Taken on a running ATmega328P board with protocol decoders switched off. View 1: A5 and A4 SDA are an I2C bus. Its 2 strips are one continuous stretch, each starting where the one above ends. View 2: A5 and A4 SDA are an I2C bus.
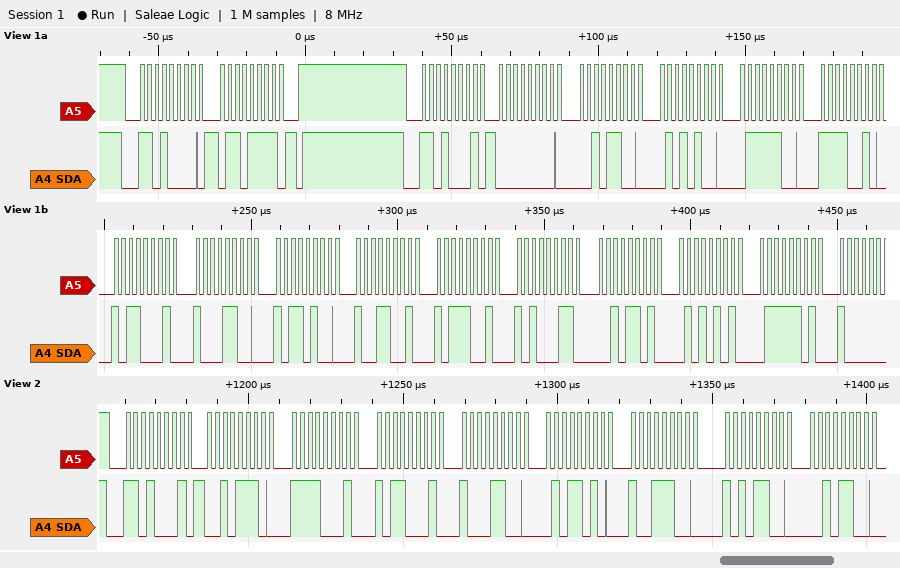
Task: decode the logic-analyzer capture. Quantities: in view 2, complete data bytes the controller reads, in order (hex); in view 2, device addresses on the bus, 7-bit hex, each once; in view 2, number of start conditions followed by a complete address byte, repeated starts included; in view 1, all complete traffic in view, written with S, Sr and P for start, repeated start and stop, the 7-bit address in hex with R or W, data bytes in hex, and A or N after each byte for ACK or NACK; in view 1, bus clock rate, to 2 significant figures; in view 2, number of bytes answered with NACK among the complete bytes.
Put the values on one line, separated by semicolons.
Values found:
2E F1 B1 8C 5A 9C AC 2C; 0x68; 1; S 68W A 6F A P S 68R A 00 A 2C A 54 A 7C A F2 A B1 A 8C A B4 A 99 A B9 A A3 A 2D A 55 A 7D A; 400 kHz; 0
